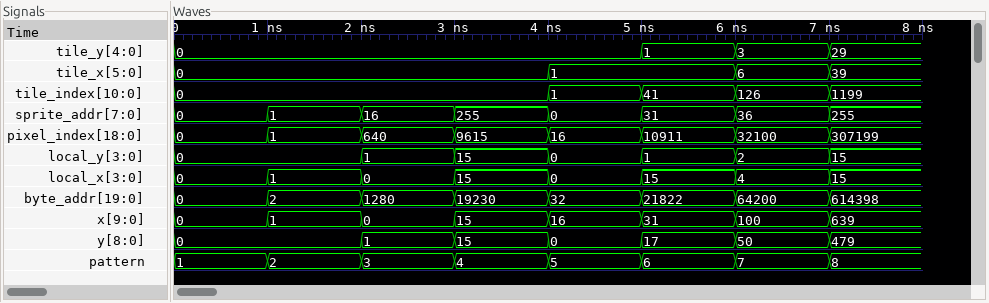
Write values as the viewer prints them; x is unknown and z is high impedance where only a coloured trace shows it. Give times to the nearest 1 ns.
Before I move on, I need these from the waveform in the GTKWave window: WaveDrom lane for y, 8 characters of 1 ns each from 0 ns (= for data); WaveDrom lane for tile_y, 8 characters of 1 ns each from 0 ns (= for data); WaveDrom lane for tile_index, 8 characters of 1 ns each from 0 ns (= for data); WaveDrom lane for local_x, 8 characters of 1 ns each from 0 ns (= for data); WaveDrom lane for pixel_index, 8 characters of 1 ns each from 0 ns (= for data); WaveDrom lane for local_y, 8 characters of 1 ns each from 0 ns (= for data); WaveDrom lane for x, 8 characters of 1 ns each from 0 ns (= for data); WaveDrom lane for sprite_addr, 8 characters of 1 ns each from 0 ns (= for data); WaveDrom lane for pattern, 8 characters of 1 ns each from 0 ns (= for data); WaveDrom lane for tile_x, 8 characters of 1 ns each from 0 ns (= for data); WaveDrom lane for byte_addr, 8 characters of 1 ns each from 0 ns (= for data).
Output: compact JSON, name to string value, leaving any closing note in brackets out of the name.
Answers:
{"WaveDrom lane for y, 8 characters of 1 ns each from 0 ns": "{name: 'y', wave: '=.======', data: '0 1 15 0 17 50 479'}", "WaveDrom lane for tile_y, 8 characters of 1 ns each from 0 ns": "{name: 'tile_y', wave: '=....===', data: '0 1 3 29'}", "WaveDrom lane for tile_index, 8 characters of 1 ns each from 0 ns": "{name: 'tile_index', wave: '=...====', data: '0 1 41 126 1199'}", "WaveDrom lane for local_x, 8 characters of 1 ns each from 0 ns": "{name: 'local_x', wave: '========', data: '0 1 0 15 0 15 4 15'}", "WaveDrom lane for pixel_index, 8 characters of 1 ns each from 0 ns": "{name: 'pixel_index', wave: '========', data: '0 1 640 9615 16 10911 32100 307199'}", "WaveDrom lane for local_y, 8 characters of 1 ns each from 0 ns": "{name: 'local_y', wave: '=.======', data: '0 1 15 0 1 2 15'}", "WaveDrom lane for x, 8 characters of 1 ns each from 0 ns": "{name: 'x', wave: '========', data: '0 1 0 15 16 31 100 639'}", "WaveDrom lane for sprite_addr, 8 characters of 1 ns each from 0 ns": "{name: 'sprite_addr', wave: '========', data: '0 1 16 255 0 31 36 255'}", "WaveDrom lane for pattern, 8 characters of 1 ns each from 0 ns": "{name: 'pattern', wave: '========', data: '1 2 3 4 5 6 7 8'}", "WaveDrom lane for tile_x, 8 characters of 1 ns each from 0 ns": "{name: 'tile_x', wave: '=...=.==', data: '0 1 6 39'}", "WaveDrom lane for byte_addr, 8 characters of 1 ns each from 0 ns": "{name: 'byte_addr', wave: '========', data: '0 2 1280 19230 32 21822 64200 614398'}"}
